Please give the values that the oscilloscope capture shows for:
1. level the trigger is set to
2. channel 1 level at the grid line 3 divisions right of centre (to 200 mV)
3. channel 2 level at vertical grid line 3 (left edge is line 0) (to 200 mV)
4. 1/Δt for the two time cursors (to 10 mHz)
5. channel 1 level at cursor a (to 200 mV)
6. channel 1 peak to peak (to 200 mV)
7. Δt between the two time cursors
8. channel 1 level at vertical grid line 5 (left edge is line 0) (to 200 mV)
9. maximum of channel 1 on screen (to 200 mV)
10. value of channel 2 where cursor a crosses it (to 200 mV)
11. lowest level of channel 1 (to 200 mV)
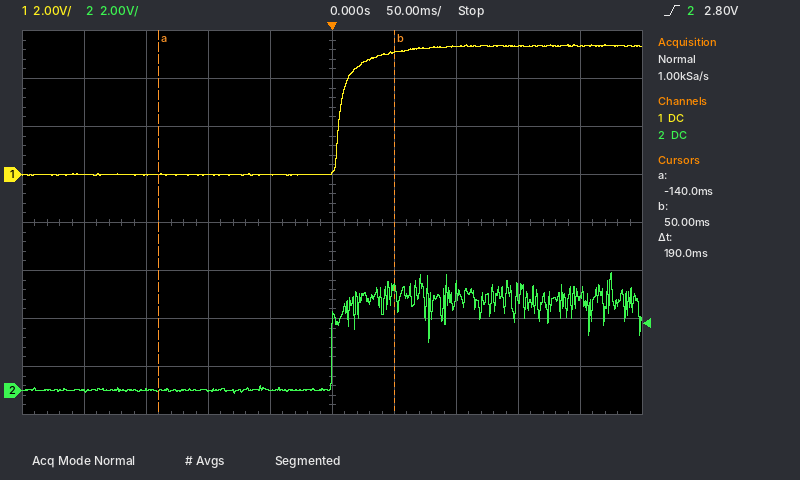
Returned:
2.80 V
5.4 V
0.0 V
5.26 Hz
0.0 V
5.4 V
190 ms
200 mV
5.4 V
0.0 V
0.0 V
